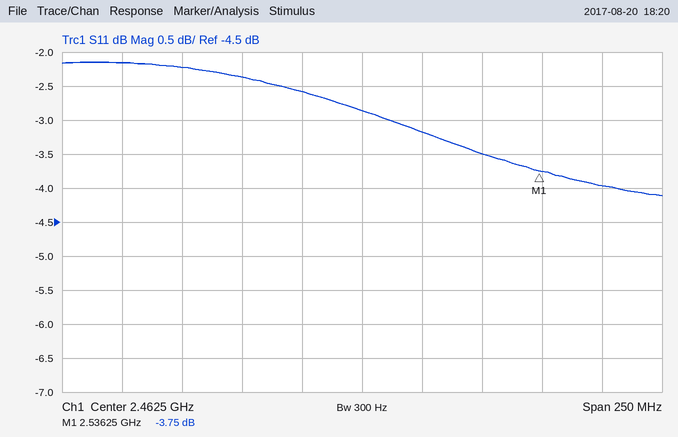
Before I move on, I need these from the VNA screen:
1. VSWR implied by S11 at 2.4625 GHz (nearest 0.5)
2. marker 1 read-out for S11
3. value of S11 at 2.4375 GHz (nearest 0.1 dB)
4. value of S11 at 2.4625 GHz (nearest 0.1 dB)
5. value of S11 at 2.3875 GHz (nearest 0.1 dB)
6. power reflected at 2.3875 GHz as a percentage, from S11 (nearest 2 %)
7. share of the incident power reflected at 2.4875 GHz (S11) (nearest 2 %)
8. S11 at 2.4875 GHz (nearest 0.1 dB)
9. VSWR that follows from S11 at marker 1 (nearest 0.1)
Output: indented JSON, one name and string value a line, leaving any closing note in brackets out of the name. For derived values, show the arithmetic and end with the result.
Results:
{
  "VSWR implied by S11 at 2.4625 GHz": "|Γ| = 10^(-2.9/20) = 0.7161; VSWR = (1 + 0.7161)/(1 − 0.7161) ≈ 6.0",
  "marker 1 read-out for S11": "-3.75 dB",
  "value of S11 at 2.4375 GHz": "-2.6 dB",
  "value of S11 at 2.4625 GHz": "-2.9 dB",
  "value of S11 at 2.3875 GHz": "-2.2 dB",
  "power reflected at 2.3875 GHz as a percentage, from S11": "10^(-2.2/10) ≈ 60 %",
  "share of the incident power reflected at 2.4875 GHz (S11)": "10^(-3.2/10) ≈ 48 %",
  "S11 at 2.4875 GHz": "-3.2 dB",
  "VSWR that follows from S11 at marker 1": "(1 + 0.6494)/(1 − 0.6494) ≈ 4.7"
}
